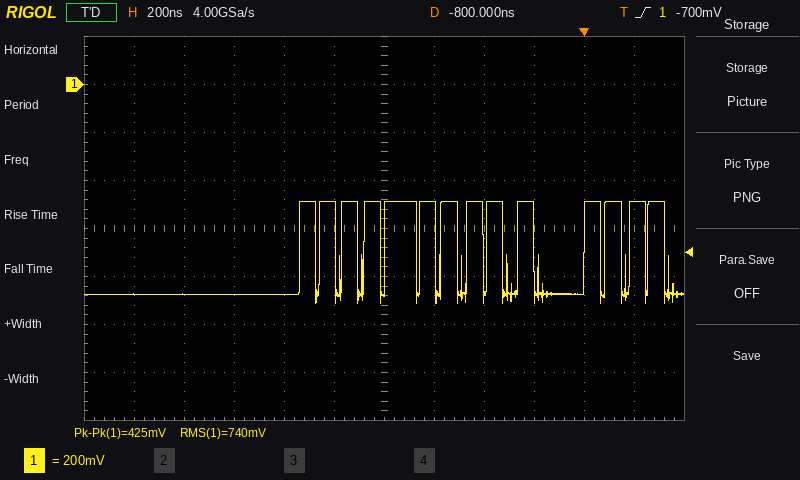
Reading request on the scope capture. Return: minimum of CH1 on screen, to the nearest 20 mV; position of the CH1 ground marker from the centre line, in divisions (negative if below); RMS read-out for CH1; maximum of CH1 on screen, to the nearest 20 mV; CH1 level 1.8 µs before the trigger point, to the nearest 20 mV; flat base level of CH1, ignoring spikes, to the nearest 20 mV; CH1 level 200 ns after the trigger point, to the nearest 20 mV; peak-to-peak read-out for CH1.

-920 mV
+3.0 div
740 mV
-480 mV
-880 mV
-880 mV
-480 mV
425 mV
